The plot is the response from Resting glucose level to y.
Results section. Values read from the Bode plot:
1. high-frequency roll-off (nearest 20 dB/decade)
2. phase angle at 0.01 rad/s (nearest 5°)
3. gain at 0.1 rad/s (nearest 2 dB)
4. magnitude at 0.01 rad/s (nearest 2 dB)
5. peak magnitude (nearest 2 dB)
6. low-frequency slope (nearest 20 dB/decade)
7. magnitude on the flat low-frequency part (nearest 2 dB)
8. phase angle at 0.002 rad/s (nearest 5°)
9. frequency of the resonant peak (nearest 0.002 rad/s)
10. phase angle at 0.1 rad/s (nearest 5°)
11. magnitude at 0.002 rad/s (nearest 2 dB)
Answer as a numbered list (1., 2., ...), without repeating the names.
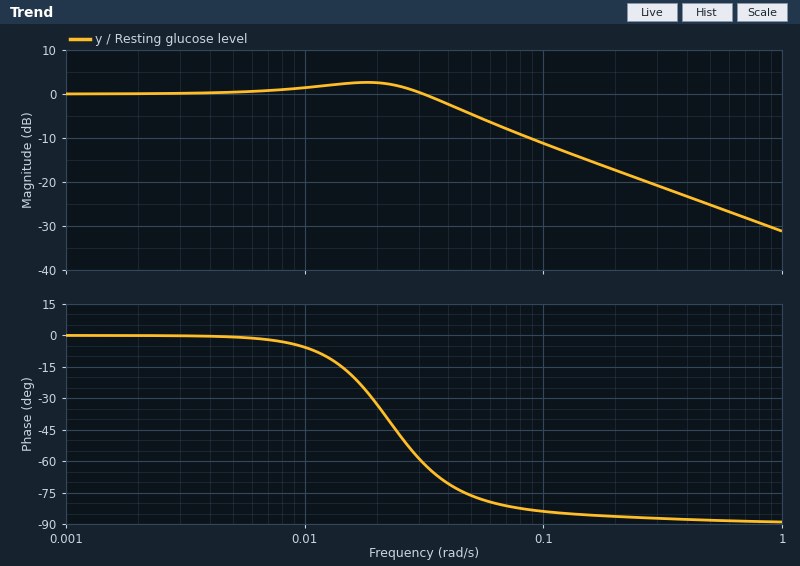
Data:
1. -20 dB/decade
2. -5°
3. -12 dB
4. 2 dB
5. 2 dB
6. 0 dB/decade
7. 0 dB
8. 0°
9. 0.018 rad/s
10. -85°
11. 0 dB
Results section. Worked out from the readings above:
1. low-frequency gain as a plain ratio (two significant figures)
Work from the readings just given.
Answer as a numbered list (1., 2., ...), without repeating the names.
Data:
1. 1.0
